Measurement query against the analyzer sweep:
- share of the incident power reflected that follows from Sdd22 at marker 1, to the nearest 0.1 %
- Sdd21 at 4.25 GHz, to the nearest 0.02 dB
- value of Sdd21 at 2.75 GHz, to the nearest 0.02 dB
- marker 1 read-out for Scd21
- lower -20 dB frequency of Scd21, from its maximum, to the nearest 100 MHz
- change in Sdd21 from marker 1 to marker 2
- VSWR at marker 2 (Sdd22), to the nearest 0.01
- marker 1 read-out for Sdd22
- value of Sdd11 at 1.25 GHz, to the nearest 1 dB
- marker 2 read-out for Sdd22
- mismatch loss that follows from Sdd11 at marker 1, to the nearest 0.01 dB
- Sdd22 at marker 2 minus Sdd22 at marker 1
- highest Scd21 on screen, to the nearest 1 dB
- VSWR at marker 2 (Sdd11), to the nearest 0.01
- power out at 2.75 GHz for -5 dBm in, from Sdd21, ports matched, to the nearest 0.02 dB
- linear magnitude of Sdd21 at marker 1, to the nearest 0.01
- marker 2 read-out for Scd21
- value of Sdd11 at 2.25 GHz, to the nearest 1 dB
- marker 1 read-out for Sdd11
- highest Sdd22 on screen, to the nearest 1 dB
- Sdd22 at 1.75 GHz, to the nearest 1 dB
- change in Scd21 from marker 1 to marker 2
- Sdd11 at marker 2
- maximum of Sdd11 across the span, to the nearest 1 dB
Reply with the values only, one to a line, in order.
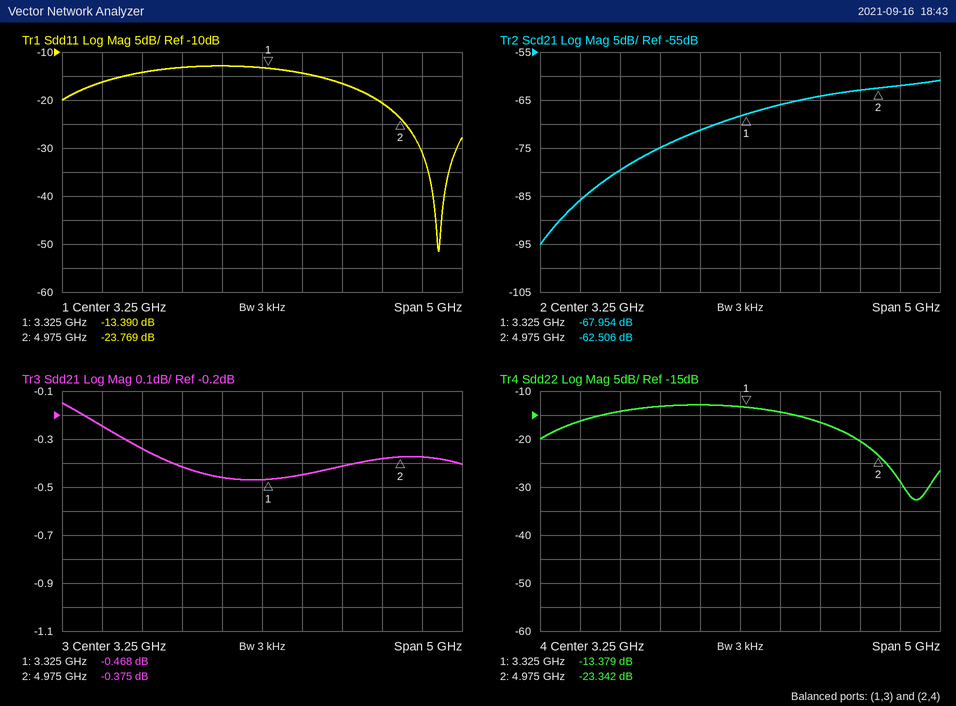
4.6 %
-0.42 dB
-0.46 dB
-67.954 dB
1.6 GHz
0.093 dB
1.15
-13.379 dB
-16 dB
-23.342 dB
0.20 dB
-9.963 dB
-61 dB
1.14
-5.46 dBm
0.95
-62.506 dB
-13 dB
-13.390 dB
-13 dB
-14 dB
5.448 dB
-23.769 dB
-13 dB
